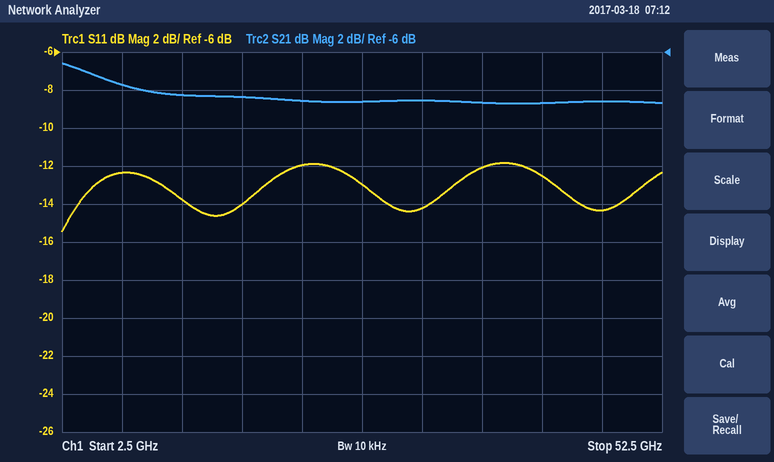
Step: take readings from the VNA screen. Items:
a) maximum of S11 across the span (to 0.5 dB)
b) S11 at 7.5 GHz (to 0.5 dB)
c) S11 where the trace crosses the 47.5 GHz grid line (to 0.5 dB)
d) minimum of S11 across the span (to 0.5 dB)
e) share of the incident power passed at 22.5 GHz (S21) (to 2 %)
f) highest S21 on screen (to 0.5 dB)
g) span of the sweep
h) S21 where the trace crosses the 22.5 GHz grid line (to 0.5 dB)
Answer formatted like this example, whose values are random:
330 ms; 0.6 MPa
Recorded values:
-12.0 dB; -12.5 dB; -14.5 dB; -15.5 dB; 14 %; -6.5 dB; 50 GHz; -8.5 dB
